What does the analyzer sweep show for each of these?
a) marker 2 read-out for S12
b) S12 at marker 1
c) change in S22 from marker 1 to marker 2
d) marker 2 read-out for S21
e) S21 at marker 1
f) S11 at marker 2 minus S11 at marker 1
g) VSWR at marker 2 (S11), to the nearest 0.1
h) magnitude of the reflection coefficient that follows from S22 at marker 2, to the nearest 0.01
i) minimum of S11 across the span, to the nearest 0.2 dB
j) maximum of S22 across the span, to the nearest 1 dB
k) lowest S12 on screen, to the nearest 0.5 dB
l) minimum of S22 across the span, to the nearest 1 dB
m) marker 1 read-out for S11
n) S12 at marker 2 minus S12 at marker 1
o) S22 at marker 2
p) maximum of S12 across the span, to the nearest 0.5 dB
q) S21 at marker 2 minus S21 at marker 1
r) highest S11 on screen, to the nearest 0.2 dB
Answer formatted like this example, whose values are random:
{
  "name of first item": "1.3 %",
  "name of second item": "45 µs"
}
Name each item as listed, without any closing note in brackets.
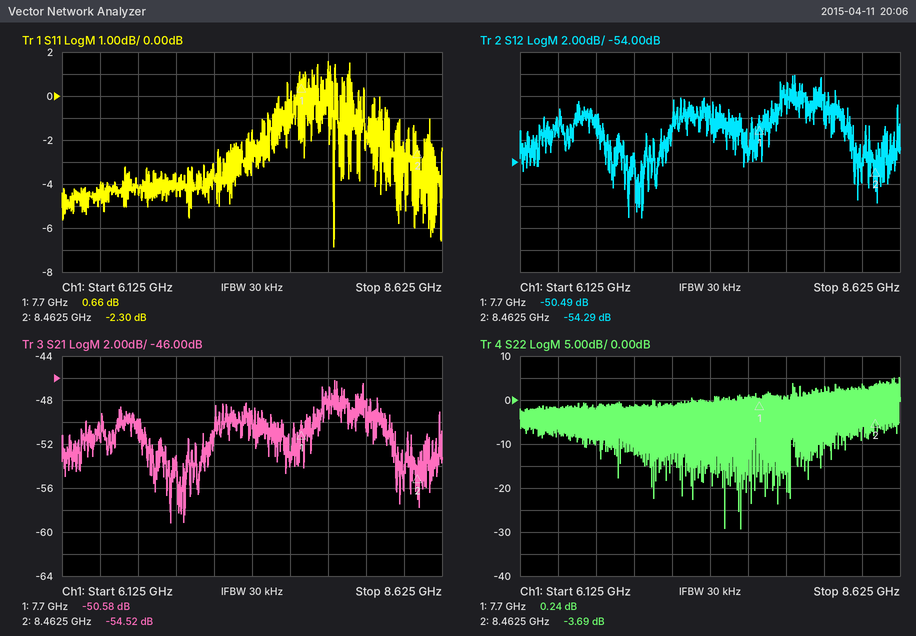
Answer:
{
  "marker 2 read-out for S12": "-54.29 dB",
  "S12 at marker 1": "-50.49 dB",
  "change in S22 from marker 1 to marker 2": "-3.93 dB",
  "marker 2 read-out for S21": "-54.52 dB",
  "S21 at marker 1": "-50.58 dB",
  "S11 at marker 2 minus S11 at marker 1": "-2.96 dB",
  "VSWR at marker 2 (S11), to the nearest 0.1": "7.6",
  "magnitude of the reflection coefficient that follows from S22 at marker 2, to the nearest 0.01": "0.65",
  "minimum of S11 across the span, to the nearest 0.2 dB": "-6.8 dB",
  "maximum of S22 across the span, to the nearest 1 dB": "5 dB",
  "lowest S12 on screen, to the nearest 0.5 dB": "-59.0 dB",
  "minimum of S22 across the span, to the nearest 1 dB": "-29 dB",
  "marker 1 read-out for S11": "0.66 dB",
  "S12 at marker 2 minus S12 at marker 1": "-3.80 dB",
  "S22 at marker 2": "-3.69 dB",
  "maximum of S12 across the span, to the nearest 0.5 dB": "-46.0 dB",
  "S21 at marker 2 minus S21 at marker 1": "-3.94 dB",
  "highest S11 on screen, to the nearest 0.2 dB": "1.6 dB"
}
